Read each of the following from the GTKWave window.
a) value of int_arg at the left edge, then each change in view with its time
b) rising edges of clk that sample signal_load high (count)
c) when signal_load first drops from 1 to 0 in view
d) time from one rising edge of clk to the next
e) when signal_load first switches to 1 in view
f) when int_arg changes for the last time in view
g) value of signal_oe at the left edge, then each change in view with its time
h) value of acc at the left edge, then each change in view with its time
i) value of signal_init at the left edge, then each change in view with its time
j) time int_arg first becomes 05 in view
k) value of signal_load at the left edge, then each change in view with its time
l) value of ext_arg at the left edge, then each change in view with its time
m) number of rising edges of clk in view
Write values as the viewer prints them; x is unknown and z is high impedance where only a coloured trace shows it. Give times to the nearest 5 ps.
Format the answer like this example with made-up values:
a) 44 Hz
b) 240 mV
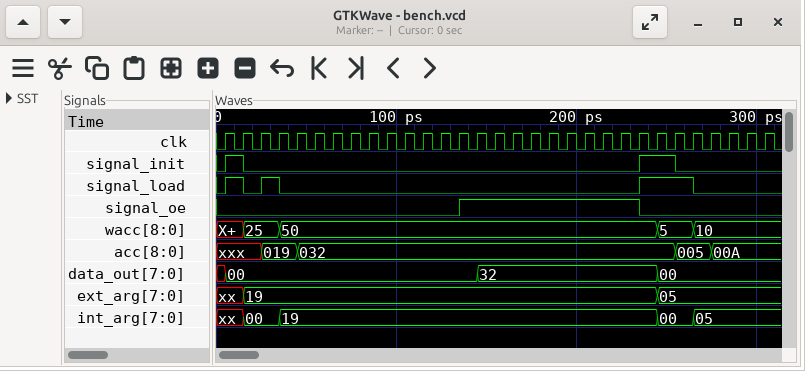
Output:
a) xx, 00 at 15 ps, 19 at 35 ps, 00 at 245 ps, 05 at 265 ps
b) 5
c) 15 ps
d) 10 ps
e) 5 ps
f) 265 ps
g) 0, 1 at 135 ps, 0 at 235 ps
h) xxx, 019 at 25 ps, 032 at 45 ps, 005 at 255 ps, 00A at 275 ps
i) 0, 1 at 5 ps, 0 at 15 ps, 1 at 235 ps, 0 at 255 ps
j) 265 ps
k) 0, 1 at 5 ps, 0 at 15 ps, 1 at 25 ps, 0 at 35 ps, 1 at 235 ps, 0 at 265 ps
l) xx, 19 at 15 ps, 05 at 245 ps
m) 31
